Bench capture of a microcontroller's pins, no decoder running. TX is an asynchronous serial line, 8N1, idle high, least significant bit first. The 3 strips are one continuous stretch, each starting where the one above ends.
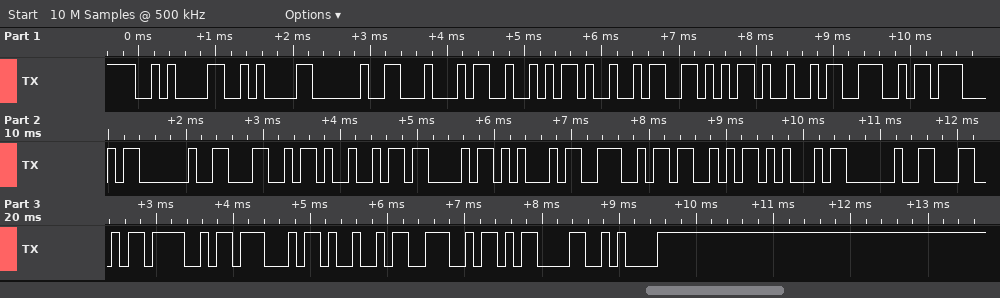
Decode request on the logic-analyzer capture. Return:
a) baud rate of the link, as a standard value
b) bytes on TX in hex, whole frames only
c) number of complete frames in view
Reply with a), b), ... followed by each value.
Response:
a) 9600 baud
b) 0A 0A 20 44 52 49 56 49 4E 47 20 4C 49 43 45 4E 53 45 20 4C 4F 47 49 4E 0D 0A
c) 26
